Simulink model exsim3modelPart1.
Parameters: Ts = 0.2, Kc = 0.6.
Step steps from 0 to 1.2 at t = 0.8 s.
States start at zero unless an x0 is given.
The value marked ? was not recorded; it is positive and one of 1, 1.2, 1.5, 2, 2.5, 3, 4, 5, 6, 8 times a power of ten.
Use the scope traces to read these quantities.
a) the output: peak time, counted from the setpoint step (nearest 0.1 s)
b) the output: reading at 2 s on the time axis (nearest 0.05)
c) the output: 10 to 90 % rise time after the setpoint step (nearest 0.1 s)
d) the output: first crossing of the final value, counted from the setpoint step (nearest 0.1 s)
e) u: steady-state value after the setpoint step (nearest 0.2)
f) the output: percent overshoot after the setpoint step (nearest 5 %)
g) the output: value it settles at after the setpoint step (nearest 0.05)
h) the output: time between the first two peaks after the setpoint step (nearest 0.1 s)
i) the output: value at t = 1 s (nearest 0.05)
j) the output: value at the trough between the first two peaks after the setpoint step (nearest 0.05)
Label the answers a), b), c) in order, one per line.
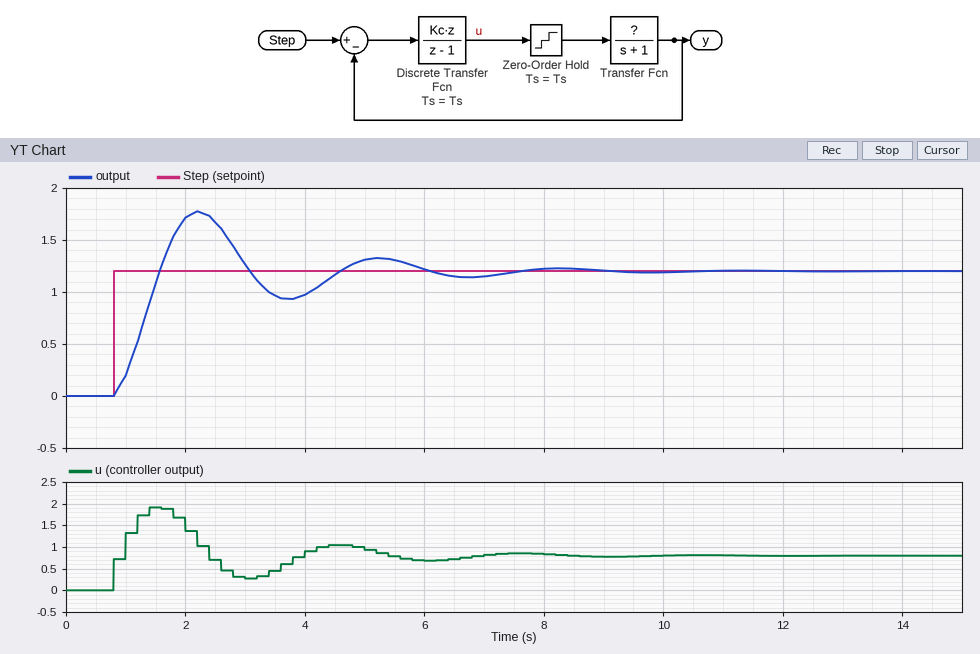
a) 1.4 s
b) 1.70
c) 0.6 s
d) 0.8 s
e) 0.8
f) 50 %
g) 1.20
h) 3.0 s
i) 0.20
j) 0.95
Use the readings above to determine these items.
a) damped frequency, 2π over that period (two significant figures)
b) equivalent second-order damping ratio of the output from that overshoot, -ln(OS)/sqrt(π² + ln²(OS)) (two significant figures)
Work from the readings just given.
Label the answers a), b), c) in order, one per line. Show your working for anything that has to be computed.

a) 2π / 3 = 2.1 rad/s
b) ln(0.5) = -0.693; 0.693 / sqrt(9.870 + 0.480) = 0.22
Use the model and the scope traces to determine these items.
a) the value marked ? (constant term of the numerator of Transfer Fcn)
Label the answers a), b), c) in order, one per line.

a) 1.5
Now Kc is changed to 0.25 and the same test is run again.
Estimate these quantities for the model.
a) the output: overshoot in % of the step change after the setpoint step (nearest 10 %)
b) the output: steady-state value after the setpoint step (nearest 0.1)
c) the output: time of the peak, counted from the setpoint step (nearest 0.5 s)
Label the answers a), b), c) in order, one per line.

a) 30 %
b) 1.2
c) 2.5 s
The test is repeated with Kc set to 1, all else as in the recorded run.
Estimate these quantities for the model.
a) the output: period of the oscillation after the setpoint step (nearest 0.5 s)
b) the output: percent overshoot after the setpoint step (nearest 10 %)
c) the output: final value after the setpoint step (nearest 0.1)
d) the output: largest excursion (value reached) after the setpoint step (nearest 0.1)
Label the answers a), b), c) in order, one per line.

a) 2.5 s
b) 60 %
c) 1.2
d) 1.9
